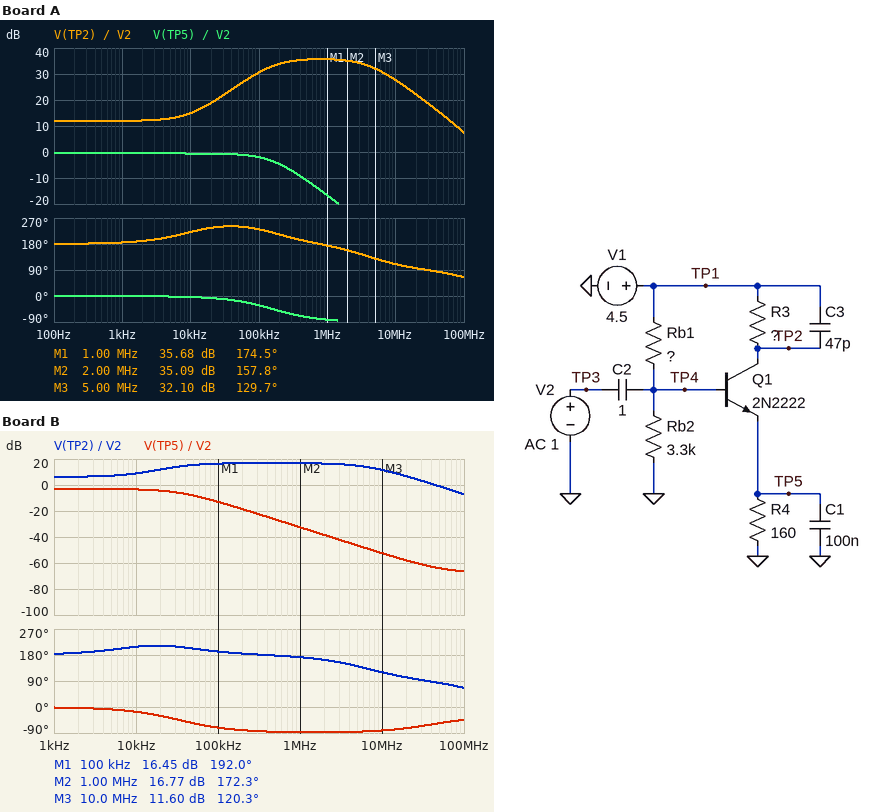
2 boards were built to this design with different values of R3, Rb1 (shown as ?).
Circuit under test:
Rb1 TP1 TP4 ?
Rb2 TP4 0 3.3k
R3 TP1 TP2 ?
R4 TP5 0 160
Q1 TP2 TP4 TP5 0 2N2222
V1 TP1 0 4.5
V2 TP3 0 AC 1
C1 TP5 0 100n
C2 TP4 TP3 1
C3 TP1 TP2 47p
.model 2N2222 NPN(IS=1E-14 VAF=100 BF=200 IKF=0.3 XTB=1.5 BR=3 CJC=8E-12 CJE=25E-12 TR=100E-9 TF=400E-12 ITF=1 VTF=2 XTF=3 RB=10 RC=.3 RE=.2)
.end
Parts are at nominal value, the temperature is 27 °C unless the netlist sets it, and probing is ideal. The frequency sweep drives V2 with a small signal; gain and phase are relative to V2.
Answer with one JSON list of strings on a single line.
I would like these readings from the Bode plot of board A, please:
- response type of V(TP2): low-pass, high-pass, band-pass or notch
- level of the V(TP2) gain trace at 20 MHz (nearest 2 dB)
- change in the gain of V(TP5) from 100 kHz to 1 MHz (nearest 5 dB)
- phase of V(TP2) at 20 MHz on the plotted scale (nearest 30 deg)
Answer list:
["band-pass", "22 dB", "-15 dB", "90 deg"]
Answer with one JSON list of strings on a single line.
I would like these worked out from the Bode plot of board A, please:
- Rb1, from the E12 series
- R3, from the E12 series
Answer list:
["10 kΩ", "680 Ω"]
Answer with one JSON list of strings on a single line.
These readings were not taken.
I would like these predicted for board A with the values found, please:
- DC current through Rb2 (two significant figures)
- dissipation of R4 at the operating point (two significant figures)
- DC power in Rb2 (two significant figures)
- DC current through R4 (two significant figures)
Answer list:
["330 µA", "1.0 mW", "360 µW", "2.5 mA"]
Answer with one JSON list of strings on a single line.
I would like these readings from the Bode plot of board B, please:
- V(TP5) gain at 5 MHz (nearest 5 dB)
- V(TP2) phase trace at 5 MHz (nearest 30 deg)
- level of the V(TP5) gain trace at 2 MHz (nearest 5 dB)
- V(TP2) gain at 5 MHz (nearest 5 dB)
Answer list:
["-45 dB", "150 deg", "-40 dB", "15 dB"]
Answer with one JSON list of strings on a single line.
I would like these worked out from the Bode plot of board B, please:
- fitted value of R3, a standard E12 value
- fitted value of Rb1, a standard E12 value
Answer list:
["470 Ω", "18 kΩ"]
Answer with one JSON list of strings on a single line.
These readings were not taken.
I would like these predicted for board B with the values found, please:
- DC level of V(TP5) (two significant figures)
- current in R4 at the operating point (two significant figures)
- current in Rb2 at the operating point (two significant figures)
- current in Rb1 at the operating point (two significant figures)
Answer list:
["62 mV", "390 µA", "210 µA", "210 µA"]
